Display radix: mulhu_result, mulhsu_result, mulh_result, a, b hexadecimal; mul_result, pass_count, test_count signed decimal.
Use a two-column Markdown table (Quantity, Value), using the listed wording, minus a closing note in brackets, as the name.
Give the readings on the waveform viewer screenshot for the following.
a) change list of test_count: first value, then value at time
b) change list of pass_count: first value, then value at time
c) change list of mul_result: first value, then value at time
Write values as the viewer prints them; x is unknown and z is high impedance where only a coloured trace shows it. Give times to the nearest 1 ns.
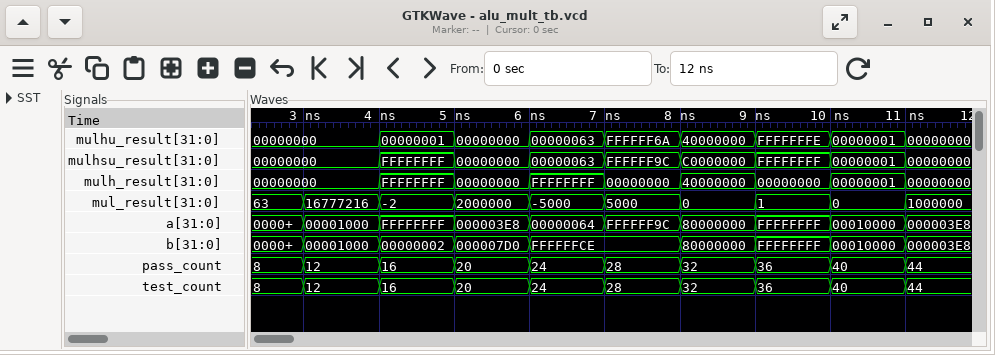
| Quantity | Value |
|---|---|
| change list of test_count: first value, then value at time | 8, 12 at 3 ns, 16 at 4 ns, 20 at 5 ns, 24 at 6 ns, 28 at 7 ns, 32 at 8 ns, 36 at 9 ns, 40 at 10 ns, 44 at 11 ns |
| change list of pass_count: first value, then value at time | 8, 12 at 3 ns, 16 at 4 ns, 20 at 5 ns, 24 at 6 ns, 28 at 7 ns, 32 at 8 ns, 36 at 9 ns, 40 at 10 ns, 44 at 11 ns |
| change list of mul_result: first value, then value at time | 63, 16777216 at 3 ns, -2 at 4 ns, 2000000 at 5 ns, -5000 at 6 ns, 5000 at 7 ns, 0 at 8 ns, 1 at 9 ns, 0 at 10 ns, 1000000 at 11 ns |
